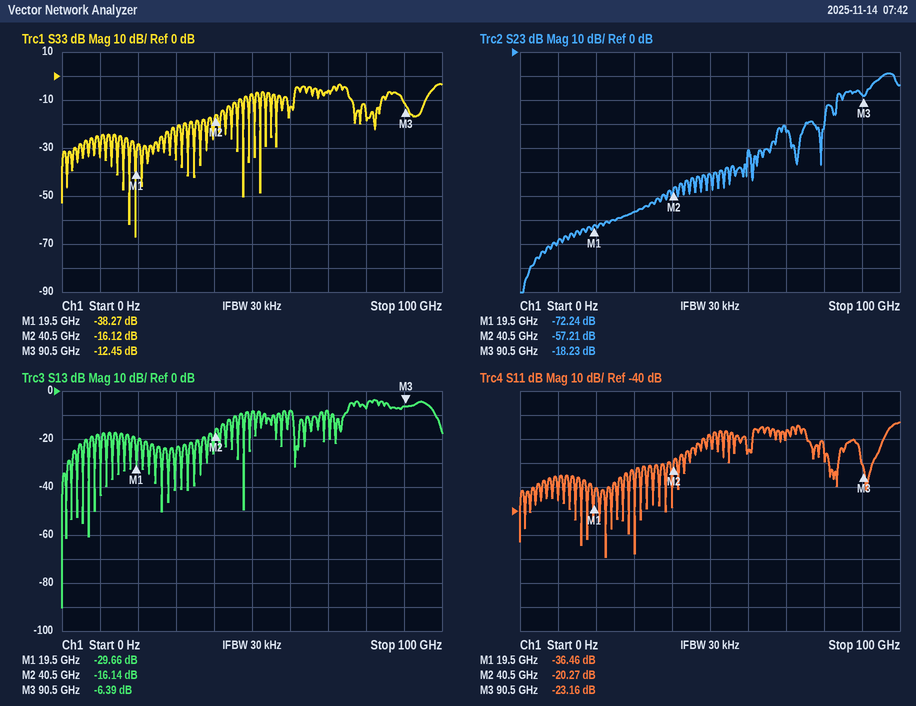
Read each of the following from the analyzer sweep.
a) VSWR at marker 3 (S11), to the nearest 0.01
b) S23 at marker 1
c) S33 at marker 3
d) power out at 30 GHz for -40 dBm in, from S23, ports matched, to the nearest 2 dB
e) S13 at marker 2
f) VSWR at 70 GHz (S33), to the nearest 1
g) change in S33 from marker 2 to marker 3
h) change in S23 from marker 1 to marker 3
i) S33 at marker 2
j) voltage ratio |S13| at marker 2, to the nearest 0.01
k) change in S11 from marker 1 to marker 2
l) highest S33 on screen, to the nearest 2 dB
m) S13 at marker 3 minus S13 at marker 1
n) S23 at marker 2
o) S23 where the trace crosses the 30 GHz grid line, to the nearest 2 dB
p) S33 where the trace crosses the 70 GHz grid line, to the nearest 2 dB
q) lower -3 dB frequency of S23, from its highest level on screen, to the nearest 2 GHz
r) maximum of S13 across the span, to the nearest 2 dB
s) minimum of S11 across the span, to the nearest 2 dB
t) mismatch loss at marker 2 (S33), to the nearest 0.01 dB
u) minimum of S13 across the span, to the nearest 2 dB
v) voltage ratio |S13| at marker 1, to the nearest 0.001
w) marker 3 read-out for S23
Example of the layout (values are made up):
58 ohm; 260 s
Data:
1.15; -72.24 dB; -12.45 dB; -106 dBm; -16.14 dB; 3; 3.67 dB; 54.01 dB; -16.12 dB; 0.16; 16.19 dB; -4 dB; 23.27 dB; -57.21 dB; -66 dB; -6 dB; 94 GHz; -4 dB; -60 dB; 0.11 dB; -90 dB; 0.033; -18.23 dB
